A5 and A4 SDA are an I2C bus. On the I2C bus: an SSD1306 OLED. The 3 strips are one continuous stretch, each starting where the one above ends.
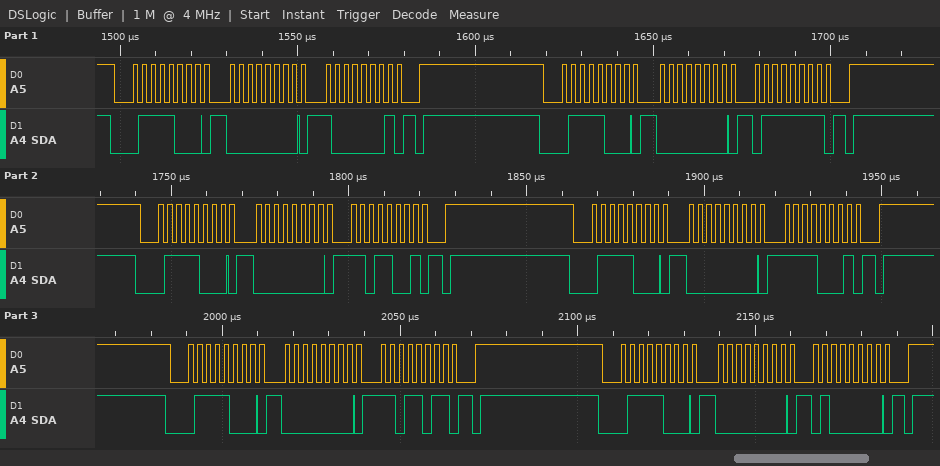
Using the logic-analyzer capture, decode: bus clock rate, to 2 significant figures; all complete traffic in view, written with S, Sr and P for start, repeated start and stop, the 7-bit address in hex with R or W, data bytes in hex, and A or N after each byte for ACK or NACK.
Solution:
400 kHz
S 3CW A 00 A 81 A P S 3CW A 00 A 7F A P S 3CW A 00 A D9 A P S 3CW A 00 A F1 A P S 3CW A 00 A DB A P S 3CW A 00 A 40 A P
